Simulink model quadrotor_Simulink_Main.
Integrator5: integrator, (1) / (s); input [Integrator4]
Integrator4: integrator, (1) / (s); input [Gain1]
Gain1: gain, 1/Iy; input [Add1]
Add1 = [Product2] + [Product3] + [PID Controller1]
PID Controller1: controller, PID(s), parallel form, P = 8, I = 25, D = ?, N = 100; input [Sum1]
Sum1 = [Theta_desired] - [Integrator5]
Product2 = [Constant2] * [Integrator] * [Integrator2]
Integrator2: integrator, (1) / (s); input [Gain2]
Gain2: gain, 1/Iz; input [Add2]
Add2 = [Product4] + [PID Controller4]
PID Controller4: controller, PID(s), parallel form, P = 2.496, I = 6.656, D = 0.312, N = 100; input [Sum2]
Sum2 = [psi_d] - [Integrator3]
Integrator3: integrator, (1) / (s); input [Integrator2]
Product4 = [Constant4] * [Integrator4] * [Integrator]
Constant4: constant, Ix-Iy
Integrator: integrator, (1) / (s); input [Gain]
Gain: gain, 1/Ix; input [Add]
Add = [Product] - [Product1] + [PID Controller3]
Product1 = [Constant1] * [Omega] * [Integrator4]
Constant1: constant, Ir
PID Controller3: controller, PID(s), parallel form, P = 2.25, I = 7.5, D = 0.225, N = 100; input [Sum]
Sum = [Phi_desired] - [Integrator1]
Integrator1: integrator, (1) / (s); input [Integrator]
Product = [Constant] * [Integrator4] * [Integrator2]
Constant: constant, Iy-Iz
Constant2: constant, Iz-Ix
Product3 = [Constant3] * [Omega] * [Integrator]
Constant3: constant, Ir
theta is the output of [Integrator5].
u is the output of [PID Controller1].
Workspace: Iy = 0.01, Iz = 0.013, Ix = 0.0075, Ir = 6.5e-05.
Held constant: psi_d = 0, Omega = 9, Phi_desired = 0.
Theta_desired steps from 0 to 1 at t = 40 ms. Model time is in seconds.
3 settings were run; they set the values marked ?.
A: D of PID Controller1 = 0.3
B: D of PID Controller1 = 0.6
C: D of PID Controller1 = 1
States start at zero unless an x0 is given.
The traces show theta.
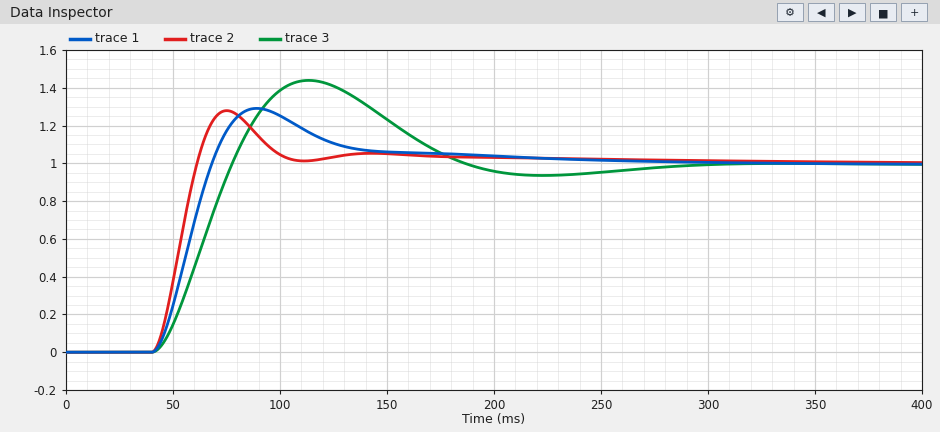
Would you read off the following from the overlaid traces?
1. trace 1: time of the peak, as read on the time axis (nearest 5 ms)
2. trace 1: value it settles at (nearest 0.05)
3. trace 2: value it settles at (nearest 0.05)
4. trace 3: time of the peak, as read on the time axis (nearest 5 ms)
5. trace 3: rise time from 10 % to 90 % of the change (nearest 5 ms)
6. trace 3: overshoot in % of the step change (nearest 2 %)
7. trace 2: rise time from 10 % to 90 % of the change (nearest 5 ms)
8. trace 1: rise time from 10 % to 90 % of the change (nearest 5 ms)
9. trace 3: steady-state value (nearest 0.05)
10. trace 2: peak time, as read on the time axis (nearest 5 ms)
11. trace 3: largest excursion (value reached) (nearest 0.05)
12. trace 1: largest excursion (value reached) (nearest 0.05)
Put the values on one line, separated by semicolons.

90 ms; 1.00; 1.00; 115 ms; 25 ms; 44 %; 15 ms; 20 ms; 1.00; 75 ms; 1.45; 1.30
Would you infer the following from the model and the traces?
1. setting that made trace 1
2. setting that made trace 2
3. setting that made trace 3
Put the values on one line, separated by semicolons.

B; C; A
